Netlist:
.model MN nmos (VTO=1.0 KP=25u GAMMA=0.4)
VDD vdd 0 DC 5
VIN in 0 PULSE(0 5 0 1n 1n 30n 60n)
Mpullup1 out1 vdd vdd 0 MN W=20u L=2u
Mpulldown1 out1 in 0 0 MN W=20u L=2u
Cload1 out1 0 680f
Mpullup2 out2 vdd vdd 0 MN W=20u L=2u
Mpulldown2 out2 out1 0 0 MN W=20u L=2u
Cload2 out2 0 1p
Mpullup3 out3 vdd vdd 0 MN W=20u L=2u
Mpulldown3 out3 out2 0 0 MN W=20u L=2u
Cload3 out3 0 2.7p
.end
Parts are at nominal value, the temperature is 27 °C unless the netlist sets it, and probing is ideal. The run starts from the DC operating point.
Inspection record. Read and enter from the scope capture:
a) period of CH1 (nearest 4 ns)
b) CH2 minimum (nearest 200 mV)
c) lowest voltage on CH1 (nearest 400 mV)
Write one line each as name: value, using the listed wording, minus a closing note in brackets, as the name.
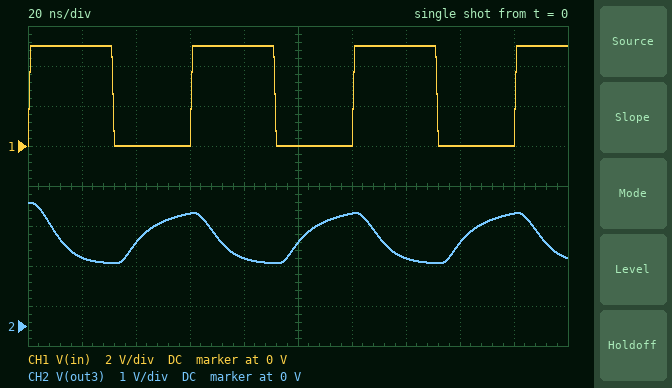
period of CH1: 60 ns
CH2 minimum: 1.6 V
lowest voltage on CH1: 0 V
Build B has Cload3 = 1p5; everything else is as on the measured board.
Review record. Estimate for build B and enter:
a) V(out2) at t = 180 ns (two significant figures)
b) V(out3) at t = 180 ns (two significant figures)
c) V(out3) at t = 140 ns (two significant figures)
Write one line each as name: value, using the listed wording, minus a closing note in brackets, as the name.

V(out2) at t = 180 ns: 1.5 V
V(out3) at t = 180 ns: 2.9 V
V(out3) at t = 140 ns: 1.6 V
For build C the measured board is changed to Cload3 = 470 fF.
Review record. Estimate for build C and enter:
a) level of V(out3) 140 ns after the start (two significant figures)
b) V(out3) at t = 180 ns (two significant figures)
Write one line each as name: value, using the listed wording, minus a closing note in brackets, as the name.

level of V(out3) 140 ns after the start: 1.6 V
V(out3) at t = 180 ns: 3.0 V
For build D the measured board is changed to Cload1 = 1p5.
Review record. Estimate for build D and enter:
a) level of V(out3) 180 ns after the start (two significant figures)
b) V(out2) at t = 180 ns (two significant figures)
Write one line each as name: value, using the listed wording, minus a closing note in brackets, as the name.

level of V(out3) 180 ns after the start: 2.7 V
V(out2) at t = 180 ns: 1.6 V
